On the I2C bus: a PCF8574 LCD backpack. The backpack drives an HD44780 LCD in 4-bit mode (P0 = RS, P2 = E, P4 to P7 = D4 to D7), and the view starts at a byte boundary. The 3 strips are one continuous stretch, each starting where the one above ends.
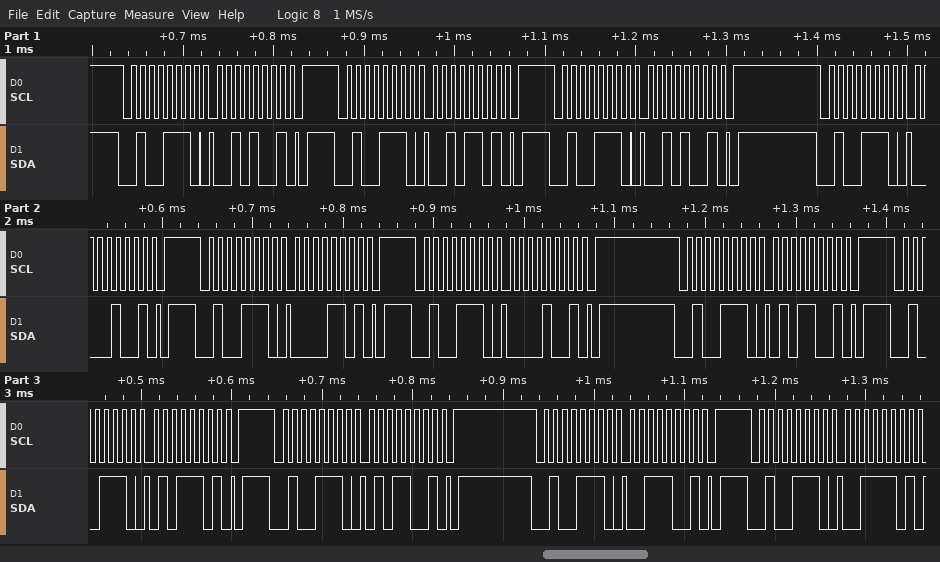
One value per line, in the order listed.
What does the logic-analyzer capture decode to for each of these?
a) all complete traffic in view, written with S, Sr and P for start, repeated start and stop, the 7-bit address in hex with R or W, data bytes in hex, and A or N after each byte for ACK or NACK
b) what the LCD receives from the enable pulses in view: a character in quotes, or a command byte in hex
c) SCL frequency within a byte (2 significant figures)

S 27W A 29 A P S 27W A 2D A P S 27W A 29 A P S 27W A 09 A P S 27W A 0D A P S 27W A 09 A P S 27W A 59 A P S 27W A 5D A P S 27W A 59 A P S 27W A 39 A P S 27W A 3D A
' '
100 kHz
